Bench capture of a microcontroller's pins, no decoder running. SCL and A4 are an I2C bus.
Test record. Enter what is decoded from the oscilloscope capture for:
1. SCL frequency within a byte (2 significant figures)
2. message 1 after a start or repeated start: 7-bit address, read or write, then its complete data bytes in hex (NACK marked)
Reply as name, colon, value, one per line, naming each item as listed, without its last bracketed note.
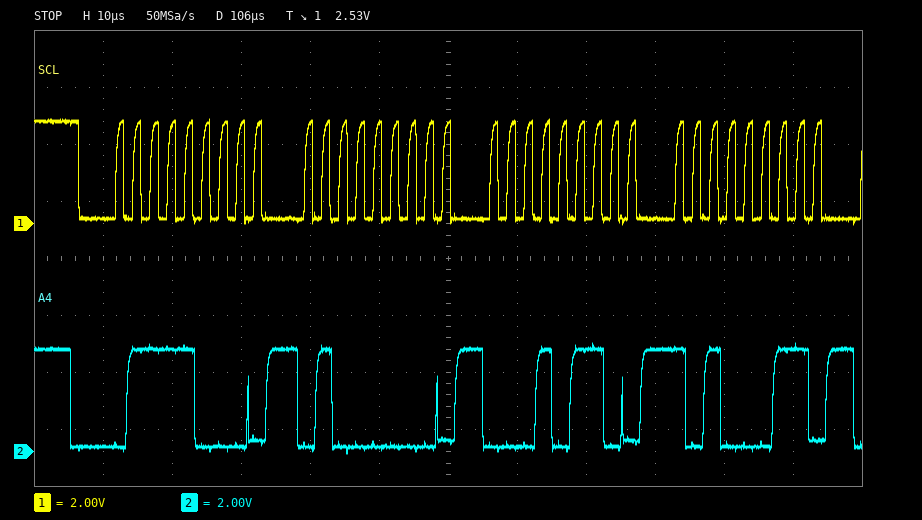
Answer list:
SCL frequency within a byte: 400 kHz
message 1 after a start or repeated start: 7-bit address, read or write, then its complete data bytes in hex: 0x3C write: 40 16 A3
